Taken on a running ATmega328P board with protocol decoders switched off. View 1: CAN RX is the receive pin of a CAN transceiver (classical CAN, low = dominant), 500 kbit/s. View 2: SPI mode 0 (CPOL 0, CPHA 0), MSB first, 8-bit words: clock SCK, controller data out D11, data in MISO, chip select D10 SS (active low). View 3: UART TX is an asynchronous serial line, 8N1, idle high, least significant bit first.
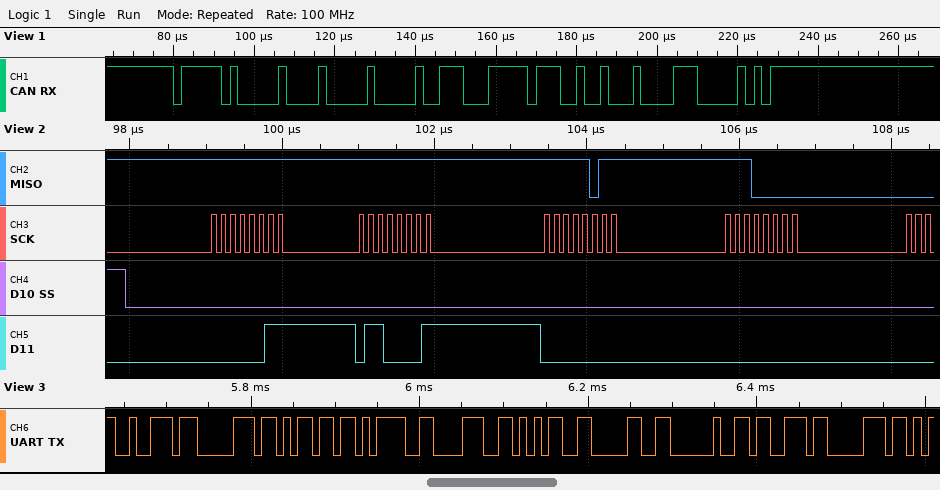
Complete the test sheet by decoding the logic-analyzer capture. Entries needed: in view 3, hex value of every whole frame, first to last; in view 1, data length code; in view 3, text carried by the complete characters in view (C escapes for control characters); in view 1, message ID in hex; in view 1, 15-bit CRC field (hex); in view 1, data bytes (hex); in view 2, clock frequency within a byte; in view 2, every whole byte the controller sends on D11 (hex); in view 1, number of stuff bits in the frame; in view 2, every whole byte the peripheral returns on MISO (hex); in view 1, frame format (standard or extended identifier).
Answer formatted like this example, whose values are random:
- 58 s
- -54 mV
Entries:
- 72 70 6D 3D 38 35 30 20 73 70
- 4
- "rpm=850 sp"
- 0x7E0
- 0x21C0
- 00 38 FF 24
- 8 MHz
- 0x03 0x61 0x00 0x00
- 6
- 0xFF 0xFF 0xFB 0xE0
- standard
